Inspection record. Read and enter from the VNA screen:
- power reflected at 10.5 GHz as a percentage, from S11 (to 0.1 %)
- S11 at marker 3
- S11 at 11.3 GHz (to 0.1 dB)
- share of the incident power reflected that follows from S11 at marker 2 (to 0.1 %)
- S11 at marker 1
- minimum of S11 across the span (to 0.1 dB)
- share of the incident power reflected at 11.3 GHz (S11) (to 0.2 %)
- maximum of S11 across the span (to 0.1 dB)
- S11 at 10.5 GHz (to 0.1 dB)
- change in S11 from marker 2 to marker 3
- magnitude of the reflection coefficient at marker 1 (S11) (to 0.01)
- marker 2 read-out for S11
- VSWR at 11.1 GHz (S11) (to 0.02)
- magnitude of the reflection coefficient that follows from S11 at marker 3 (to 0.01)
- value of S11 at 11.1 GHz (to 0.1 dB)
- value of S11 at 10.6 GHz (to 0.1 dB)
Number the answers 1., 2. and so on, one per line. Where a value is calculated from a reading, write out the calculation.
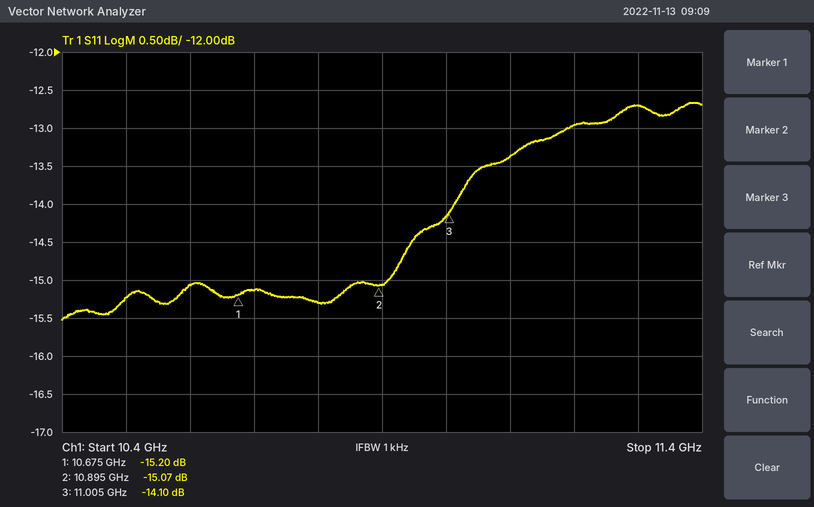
1. 10^(-15.2/10) ≈ 3.0 %
2. -14.10 dB
3. -12.7 dB
4. 10^(-15.07/10) ≈ 3.1 %
5. -15.20 dB
6. -15.5 dB
7. 10^(-12.7/10) ≈ 5.4 %
8. -12.7 dB
9. -15.2 dB
10. -14.1 − (-15.07) = 0.97 dB
11. 10^(-15.2/20) ≈ 0.17
12. -15.07 dB
13. |Γ| = 10^(-13.4/20) = 0.2138; VSWR = (1 + 0.2138)/(1 − 0.2138) ≈ 1.54
14. 10^(-14.1/20) ≈ 0.20
15. -13.4 dB
16. -15.1 dB
